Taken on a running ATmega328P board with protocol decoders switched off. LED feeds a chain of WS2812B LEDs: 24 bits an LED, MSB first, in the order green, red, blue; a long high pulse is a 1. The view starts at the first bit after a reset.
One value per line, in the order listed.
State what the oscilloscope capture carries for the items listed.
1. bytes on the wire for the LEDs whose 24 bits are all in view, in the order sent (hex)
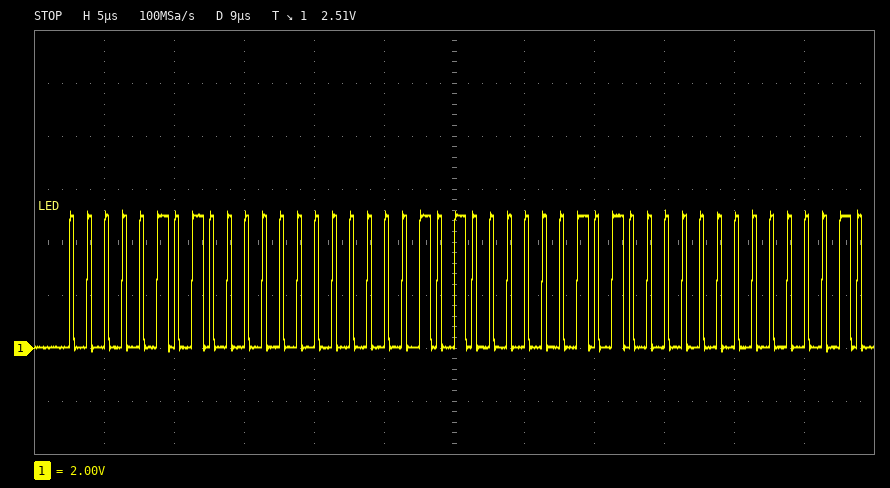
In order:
05 00 0A
